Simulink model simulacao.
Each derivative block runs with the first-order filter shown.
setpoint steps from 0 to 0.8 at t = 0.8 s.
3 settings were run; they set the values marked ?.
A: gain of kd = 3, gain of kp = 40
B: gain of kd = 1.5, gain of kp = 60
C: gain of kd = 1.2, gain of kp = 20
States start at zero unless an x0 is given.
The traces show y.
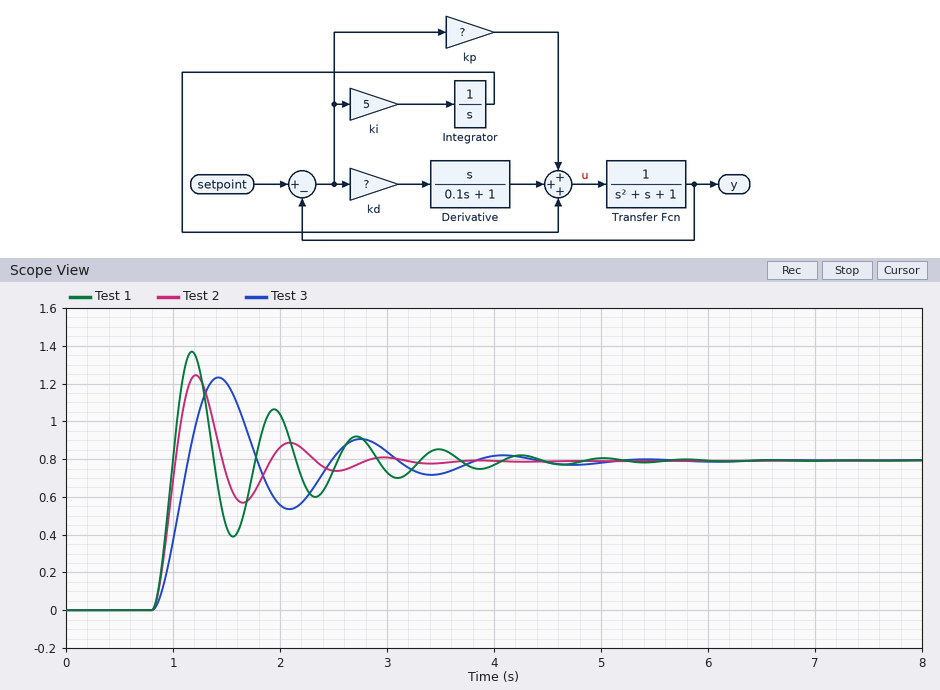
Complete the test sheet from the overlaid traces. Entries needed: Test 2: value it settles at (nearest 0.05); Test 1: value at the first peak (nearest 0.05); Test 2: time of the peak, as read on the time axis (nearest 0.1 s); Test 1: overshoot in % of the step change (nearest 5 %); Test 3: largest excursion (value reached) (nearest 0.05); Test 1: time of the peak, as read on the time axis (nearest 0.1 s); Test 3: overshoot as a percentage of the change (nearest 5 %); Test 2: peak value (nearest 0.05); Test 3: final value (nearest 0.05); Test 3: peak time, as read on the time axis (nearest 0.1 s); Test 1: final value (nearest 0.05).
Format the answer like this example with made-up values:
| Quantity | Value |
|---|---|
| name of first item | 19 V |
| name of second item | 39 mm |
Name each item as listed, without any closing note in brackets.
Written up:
| Quantity | Value |
|---|---|
| Test 2: value it settles at | 0.80 |
| Test 1: value at the first peak | 1.35 |
| Test 2: time of the peak, as read on the time axis | 1.2 s |
| Test 1: overshoot in % of the step change | 70 % |
| Test 3: largest excursion (value reached) | 1.25 |
| Test 1: time of the peak, as read on the time axis | 1.2 s |
| Test 3: overshoot as a percentage of the change | 55 % |
| Test 2: peak value | 1.25 |
| Test 3: final value | 0.80 |
| Test 3: peak time, as read on the time axis | 1.4 s |
| Test 1: final value | 0.80 |
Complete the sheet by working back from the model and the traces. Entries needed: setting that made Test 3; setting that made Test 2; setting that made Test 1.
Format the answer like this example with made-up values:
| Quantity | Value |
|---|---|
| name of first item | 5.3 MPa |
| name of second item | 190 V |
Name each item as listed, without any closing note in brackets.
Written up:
| Quantity | Value |
|---|---|
| setting that made Test 3 | C |
| setting that made Test 2 | A |
| setting that made Test 1 | B |
